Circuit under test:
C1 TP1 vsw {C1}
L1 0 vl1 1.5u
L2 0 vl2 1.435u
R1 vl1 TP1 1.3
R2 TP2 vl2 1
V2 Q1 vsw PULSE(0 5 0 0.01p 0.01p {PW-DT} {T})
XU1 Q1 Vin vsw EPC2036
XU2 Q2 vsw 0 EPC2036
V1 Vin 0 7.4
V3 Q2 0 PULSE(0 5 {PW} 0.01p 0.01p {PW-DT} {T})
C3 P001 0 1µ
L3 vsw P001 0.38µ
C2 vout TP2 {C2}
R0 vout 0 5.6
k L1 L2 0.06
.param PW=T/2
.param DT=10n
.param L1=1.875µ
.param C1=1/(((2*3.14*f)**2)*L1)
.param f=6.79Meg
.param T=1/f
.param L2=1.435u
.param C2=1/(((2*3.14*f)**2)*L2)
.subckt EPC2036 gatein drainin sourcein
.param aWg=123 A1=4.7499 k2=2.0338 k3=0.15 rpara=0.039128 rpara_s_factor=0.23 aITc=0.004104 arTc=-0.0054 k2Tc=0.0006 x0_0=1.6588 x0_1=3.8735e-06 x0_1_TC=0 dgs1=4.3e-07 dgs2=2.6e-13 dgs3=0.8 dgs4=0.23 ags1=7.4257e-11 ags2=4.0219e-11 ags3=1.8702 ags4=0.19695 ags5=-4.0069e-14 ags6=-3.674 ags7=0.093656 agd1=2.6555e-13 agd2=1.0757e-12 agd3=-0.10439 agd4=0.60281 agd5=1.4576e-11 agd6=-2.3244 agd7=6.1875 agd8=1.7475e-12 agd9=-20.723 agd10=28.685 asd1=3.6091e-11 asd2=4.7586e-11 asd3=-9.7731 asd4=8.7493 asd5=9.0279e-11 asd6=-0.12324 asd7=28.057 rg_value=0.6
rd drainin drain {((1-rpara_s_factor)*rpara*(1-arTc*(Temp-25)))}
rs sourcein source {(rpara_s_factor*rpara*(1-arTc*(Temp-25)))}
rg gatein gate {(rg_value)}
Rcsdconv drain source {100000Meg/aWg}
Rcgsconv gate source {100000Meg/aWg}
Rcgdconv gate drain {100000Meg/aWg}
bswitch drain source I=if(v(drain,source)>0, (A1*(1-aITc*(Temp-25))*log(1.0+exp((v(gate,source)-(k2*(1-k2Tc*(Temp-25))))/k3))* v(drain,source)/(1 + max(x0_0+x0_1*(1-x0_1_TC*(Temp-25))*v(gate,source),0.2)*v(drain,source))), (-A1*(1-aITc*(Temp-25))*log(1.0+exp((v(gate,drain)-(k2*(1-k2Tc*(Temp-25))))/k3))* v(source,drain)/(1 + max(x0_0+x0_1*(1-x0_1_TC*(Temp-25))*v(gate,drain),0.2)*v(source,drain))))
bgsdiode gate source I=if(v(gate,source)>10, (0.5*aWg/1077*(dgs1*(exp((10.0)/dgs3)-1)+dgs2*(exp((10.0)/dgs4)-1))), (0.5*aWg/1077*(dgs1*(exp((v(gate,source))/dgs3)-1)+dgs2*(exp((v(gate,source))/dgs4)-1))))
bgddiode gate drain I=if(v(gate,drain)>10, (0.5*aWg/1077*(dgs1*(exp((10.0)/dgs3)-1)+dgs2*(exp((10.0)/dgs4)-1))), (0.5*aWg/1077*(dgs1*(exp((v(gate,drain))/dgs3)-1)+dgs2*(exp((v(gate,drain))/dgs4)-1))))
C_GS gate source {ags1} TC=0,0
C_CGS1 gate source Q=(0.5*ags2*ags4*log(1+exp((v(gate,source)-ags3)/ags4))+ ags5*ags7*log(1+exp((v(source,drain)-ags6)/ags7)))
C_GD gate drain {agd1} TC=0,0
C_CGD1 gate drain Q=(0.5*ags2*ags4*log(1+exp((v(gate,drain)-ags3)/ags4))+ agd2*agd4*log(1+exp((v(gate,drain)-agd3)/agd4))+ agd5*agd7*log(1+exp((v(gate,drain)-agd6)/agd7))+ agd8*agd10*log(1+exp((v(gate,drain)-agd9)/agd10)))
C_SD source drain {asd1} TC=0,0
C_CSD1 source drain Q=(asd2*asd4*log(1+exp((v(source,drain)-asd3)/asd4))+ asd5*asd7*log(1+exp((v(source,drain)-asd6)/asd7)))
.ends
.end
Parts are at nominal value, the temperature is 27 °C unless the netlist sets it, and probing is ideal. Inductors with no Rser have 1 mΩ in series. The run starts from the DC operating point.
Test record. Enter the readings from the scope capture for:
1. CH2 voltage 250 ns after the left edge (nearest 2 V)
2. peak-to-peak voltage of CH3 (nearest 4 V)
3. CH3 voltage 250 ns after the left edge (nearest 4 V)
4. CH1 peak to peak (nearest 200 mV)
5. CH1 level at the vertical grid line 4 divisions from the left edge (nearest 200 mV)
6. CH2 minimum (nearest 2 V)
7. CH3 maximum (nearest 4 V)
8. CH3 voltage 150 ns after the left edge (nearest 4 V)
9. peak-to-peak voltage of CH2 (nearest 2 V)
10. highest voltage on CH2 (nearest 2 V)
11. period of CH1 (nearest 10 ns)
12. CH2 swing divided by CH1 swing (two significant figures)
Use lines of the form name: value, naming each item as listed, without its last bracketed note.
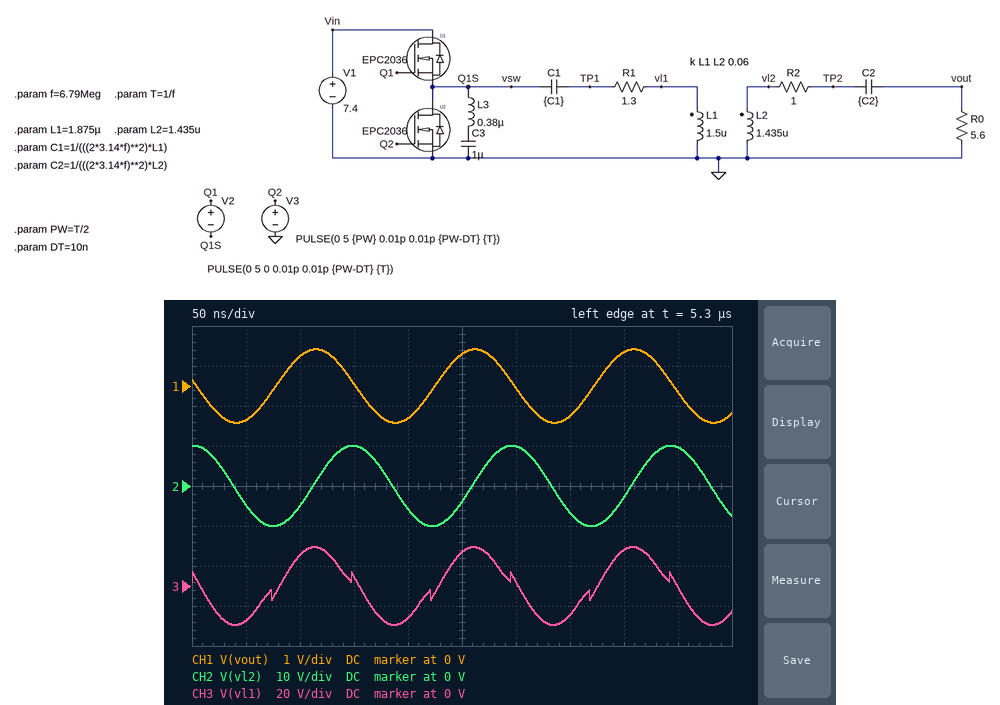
CH2 voltage 250 ns after the left edge: -4 V
peak-to-peak voltage of CH3: 40 V
CH3 voltage 250 ns after the left edge: 16 V
CH1 peak to peak: 1.8 V
CH1 level at the vertical grid line 4 divisions from the left edge: -800 mV
CH2 minimum: -10 V
CH3 maximum: 20 V
CH3 voltage 150 ns after the left edge: 4 V
peak-to-peak voltage of CH2: 20 V
highest voltage on CH2: 10 V
period of CH1: 150 ns
CH2 swing divided by CH1 swing: 11
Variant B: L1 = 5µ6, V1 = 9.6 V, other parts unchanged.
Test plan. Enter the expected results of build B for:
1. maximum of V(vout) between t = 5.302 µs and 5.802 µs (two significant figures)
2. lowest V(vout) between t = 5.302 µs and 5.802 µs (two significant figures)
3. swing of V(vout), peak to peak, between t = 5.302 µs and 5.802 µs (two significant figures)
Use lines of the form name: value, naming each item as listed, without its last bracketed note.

maximum of V(vout) between t = 5.302 µs and 5.802 µs: 240 mV
lowest V(vout) between t = 5.302 µs and 5.802 µs: -240 mV
swing of V(vout), peak to peak, between t = 5.302 µs and 5.802 µs: 480 mV
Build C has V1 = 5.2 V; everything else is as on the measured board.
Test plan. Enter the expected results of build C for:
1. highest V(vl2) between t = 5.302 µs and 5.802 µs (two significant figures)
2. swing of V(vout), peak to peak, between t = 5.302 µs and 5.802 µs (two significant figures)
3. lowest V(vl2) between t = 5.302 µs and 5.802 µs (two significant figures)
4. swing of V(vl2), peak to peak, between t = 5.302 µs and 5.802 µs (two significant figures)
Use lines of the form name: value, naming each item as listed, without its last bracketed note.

highest V(vl2) between t = 5.302 µs and 5.802 µs: 7.1 V
swing of V(vout), peak to peak, between t = 5.302 µs and 5.802 µs: 1.3 V
lowest V(vl2) between t = 5.302 µs and 5.802 µs: -7.1 V
swing of V(vl2), peak to peak, between t = 5.302 µs and 5.802 µs: 14 V
